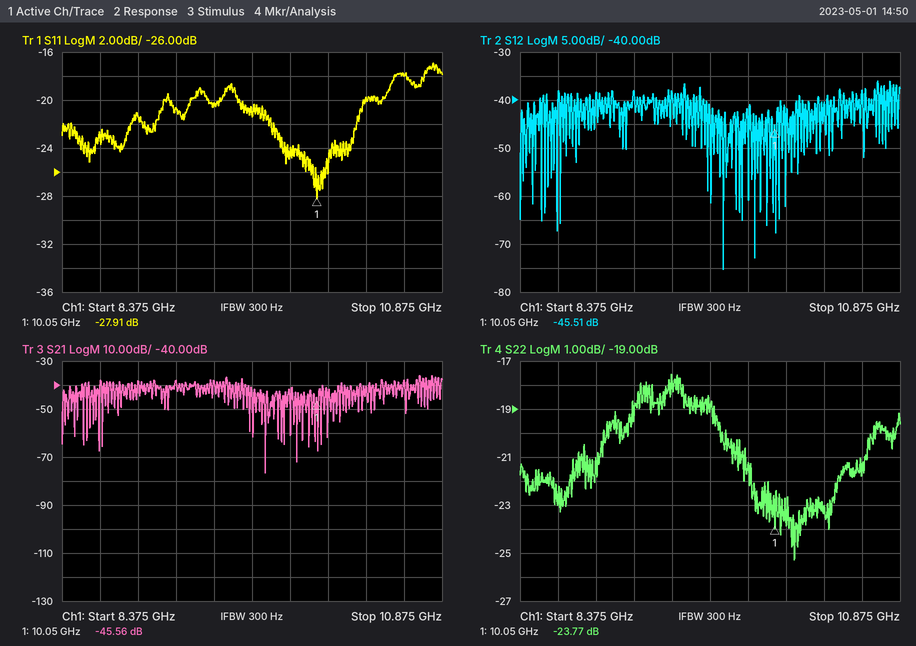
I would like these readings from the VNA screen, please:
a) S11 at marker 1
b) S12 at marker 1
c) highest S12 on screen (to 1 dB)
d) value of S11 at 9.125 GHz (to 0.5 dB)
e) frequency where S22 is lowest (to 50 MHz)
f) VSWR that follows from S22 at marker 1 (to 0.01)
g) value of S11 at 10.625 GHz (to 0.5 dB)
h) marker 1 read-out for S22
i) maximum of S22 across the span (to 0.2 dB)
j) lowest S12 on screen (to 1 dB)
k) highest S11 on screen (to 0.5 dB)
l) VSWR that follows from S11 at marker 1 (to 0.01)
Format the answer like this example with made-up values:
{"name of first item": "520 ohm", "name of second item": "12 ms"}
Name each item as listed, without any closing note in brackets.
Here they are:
{"S11 at marker 1": "-27.91 dB", "S12 at marker 1": "-45.51 dB", "highest S12 on screen": "-36 dB", "value of S11 at 9.125 GHz": "-20.5 dB", "frequency where S22 is lowest": "10.20 GHz", "VSWR that follows from S22 at marker 1": "1.14", "value of S11 at 10.625 GHz": "-18.0 dB", "marker 1 read-out for S22": "-23.77 dB", "maximum of S22 across the span": "-17.6 dB", "lowest S12 on screen": "-75 dB", "highest S11 on screen": "-17.0 dB", "VSWR that follows from S11 at marker 1": "1.08"}
